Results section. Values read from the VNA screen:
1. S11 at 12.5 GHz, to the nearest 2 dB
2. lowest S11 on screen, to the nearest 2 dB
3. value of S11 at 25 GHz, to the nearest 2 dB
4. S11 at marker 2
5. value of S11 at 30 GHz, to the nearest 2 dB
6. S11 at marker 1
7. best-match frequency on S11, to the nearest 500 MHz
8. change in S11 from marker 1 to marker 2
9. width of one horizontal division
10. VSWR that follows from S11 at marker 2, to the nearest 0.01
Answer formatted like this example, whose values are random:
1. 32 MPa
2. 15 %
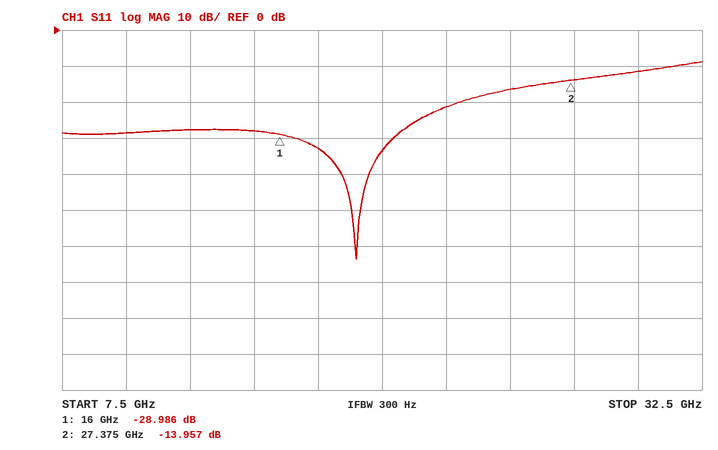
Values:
1. -28 dB
2. -64 dB
3. -16 dB
4. -13.957 dB
5. -12 dB
6. -28.986 dB
7. 19.0 GHz
8. 15.029 dB
9. 2.5 GHz
10. 1.50
